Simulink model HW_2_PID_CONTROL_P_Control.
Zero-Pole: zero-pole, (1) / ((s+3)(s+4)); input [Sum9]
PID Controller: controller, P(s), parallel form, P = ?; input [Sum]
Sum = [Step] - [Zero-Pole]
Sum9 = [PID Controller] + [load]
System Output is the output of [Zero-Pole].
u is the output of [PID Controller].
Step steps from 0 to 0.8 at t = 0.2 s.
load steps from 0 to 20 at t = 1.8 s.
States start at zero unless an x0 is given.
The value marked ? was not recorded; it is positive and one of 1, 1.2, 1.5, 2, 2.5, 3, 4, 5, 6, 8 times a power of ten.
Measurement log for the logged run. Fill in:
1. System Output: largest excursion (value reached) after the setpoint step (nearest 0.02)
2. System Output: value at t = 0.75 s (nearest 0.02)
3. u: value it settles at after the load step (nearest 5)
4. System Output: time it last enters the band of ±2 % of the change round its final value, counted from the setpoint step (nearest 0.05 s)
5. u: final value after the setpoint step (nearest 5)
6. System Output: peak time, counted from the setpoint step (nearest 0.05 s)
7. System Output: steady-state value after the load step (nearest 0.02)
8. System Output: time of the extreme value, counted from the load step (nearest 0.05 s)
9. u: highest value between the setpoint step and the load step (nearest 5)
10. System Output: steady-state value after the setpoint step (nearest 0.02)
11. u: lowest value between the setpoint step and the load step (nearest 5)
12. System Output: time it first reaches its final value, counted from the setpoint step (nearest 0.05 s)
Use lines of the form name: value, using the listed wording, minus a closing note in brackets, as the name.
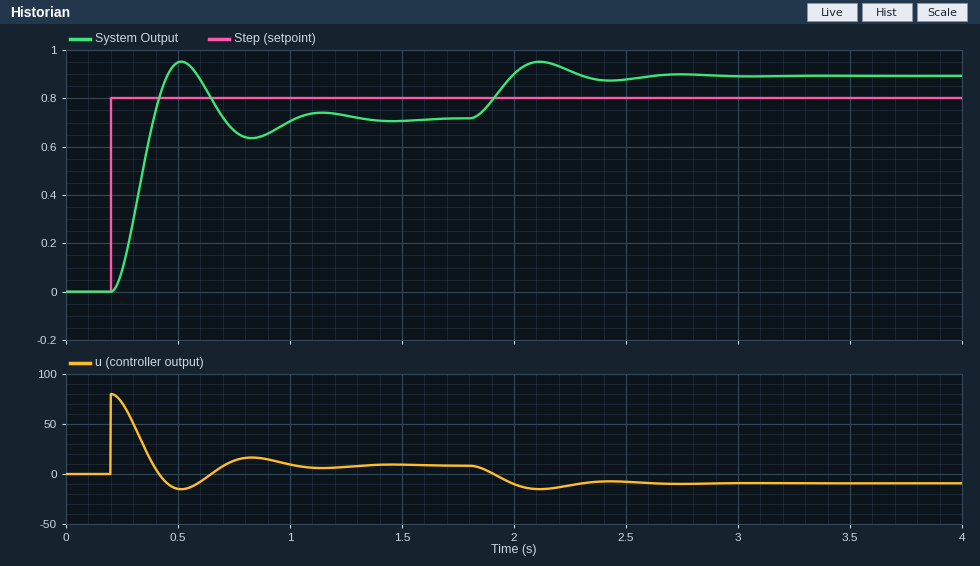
System Output: largest excursion (value reached) after the setpoint step: 0.96
System Output: value at t = 0.75 s: 0.66
u: value it settles at after the load step: -10
System Output: time it last enters the band of ±2 % of the change round its final value, counted from the setpoint step: 1.05 s
u: final value after the setpoint step: 10
System Output: peak time, counted from the setpoint step: 0.30 s
System Output: steady-state value after the load step: 0.90
System Output: time of the extreme value, counted from the load step: 0.30 s
u: highest value between the setpoint step and the load step: 80
System Output: steady-state value after the setpoint step: 0.72
u: lowest value between the setpoint step and the load step: -15
System Output: time it first reaches its final value, counted from the setpoint step: 0.20 s
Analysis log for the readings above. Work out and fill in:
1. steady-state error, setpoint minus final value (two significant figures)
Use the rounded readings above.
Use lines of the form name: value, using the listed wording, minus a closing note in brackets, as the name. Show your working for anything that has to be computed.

steady-state error, setpoint minus final value: 0.8 - 0.72 = 0.080
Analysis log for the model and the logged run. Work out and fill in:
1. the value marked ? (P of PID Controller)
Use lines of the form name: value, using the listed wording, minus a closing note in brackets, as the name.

the value marked ?: 100
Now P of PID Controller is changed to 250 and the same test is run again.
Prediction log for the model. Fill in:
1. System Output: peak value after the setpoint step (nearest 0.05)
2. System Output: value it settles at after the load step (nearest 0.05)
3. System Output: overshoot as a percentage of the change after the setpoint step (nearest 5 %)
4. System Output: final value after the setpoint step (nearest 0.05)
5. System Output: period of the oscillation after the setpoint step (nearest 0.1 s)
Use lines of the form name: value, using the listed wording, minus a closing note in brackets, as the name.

System Output: peak value after the setpoint step: 1.15
System Output: value it settles at after the load step: 0.85
System Output: overshoot as a percentage of the change after the setpoint step: 50 %
System Output: final value after the setpoint step: 0.75
System Output: period of the oscillation after the setpoint step: 0.4 s
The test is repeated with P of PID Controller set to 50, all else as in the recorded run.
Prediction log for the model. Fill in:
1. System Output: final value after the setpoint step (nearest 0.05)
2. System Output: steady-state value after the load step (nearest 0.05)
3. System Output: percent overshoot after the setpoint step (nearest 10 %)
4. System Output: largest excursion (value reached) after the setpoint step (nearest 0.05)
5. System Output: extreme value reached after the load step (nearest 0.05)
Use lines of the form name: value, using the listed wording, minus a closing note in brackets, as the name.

System Output: final value after the setpoint step: 0.65
System Output: steady-state value after the load step: 0.95
System Output: percent overshoot after the setpoint step: 20 %
System Output: largest excursion (value reached) after the setpoint step: 0.80
System Output: extreme value reached after the load step: 1.05
